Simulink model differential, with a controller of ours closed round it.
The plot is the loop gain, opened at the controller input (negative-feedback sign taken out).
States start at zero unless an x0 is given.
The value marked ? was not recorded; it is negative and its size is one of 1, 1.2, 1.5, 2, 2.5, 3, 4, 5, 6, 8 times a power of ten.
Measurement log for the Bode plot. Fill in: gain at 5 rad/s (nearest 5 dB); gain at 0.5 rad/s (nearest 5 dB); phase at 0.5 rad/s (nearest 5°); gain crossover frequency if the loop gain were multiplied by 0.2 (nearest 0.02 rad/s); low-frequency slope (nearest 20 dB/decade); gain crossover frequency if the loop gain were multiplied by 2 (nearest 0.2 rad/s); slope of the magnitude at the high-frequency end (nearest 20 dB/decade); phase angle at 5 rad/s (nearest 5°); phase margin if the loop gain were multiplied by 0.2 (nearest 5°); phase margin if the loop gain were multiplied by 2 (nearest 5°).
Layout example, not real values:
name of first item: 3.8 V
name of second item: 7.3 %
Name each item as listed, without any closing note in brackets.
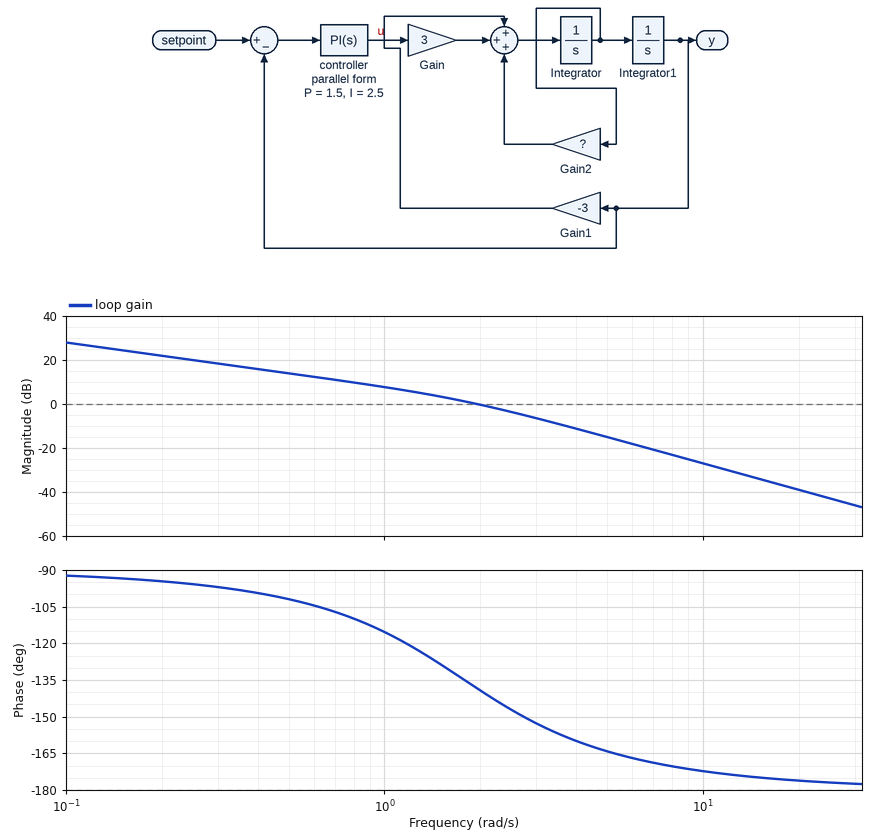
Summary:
gain at 5 rad/s: -15 dB
gain at 0.5 rad/s: 15 dB
phase at 0.5 rad/s: -100°
gain crossover frequency if the loop gain were multiplied by 0.2: 0.50 rad/s
low-frequency slope: -20 dB/decade
gain crossover frequency if the loop gain were multiplied by 2: 3.0 rad/s
slope of the magnitude at the high-frequency end: -40 dB/decade
phase angle at 5 rad/s: -165°
phase margin if the loop gain were multiplied by 0.2: 80°
phase margin if the loop gain were multiplied by 2: 30°
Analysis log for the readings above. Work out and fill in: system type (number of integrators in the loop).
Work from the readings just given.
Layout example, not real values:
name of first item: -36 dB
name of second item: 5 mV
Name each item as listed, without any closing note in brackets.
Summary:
system type: 1
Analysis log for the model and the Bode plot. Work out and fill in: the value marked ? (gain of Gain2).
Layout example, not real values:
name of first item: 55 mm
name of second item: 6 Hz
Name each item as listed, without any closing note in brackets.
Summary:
the value marked ?: -3
